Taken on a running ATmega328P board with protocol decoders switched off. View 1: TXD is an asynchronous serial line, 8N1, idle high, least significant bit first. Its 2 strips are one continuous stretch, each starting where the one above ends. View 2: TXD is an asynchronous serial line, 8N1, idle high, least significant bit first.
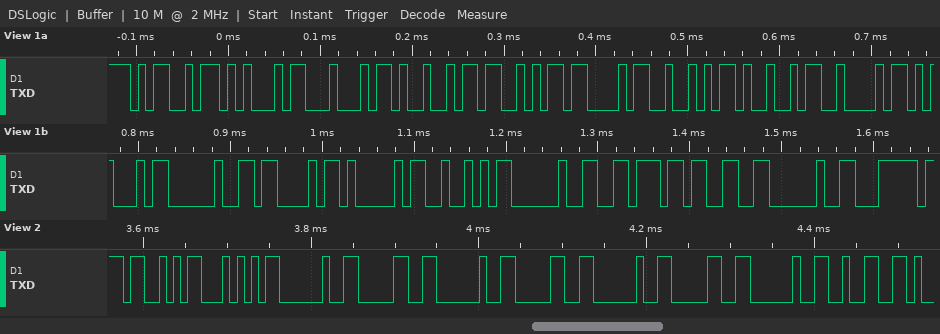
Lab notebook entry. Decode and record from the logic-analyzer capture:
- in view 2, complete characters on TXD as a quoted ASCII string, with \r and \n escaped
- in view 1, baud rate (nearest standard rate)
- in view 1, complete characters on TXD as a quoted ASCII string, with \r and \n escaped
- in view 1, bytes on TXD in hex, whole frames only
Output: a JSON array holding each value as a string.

["\"ST 0 0 0 2\"", "115200 baud", "\"MEDISCRIBE CAR v3 |\"", "0x4D 0x45 0x44 0x49 0x53 0x43 0x52 0x49 0x42 0x45 0x20 0x43 0x41 0x52 0x20 0x76 0x33 0x20 0x7C"]
